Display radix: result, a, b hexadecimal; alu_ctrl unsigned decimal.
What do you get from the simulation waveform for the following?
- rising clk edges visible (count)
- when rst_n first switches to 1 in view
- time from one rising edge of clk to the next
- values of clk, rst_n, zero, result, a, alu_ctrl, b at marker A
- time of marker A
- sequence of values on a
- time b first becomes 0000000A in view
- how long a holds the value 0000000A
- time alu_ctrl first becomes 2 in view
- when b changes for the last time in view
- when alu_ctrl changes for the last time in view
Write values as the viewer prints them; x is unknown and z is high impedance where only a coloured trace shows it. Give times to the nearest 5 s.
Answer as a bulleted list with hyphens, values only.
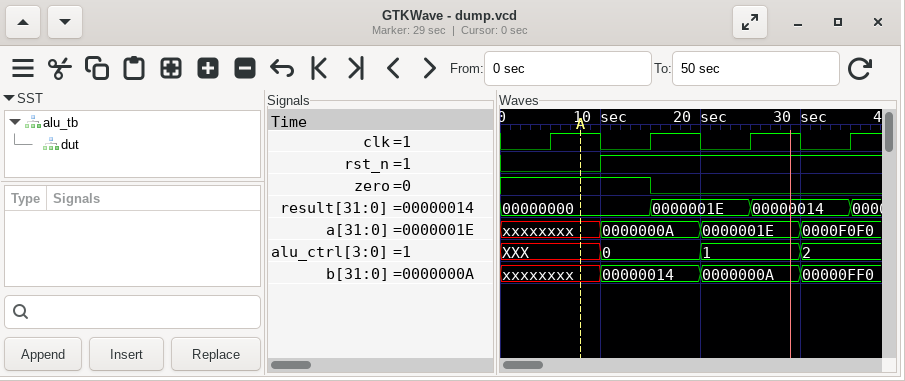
- 4
- 10 s
- 10 s
- clk=1, rst_n=0, zero=1, result=00000000, a=xxxxxxxx, alu_ctrl=XXX, b=xxxxxxxx
- 10 s
- xxxxxxxx, 0000000A, 0000001E, 0000F0F0
- 20 s
- 10 s
- 30 s
- 30 s
- 30 s
